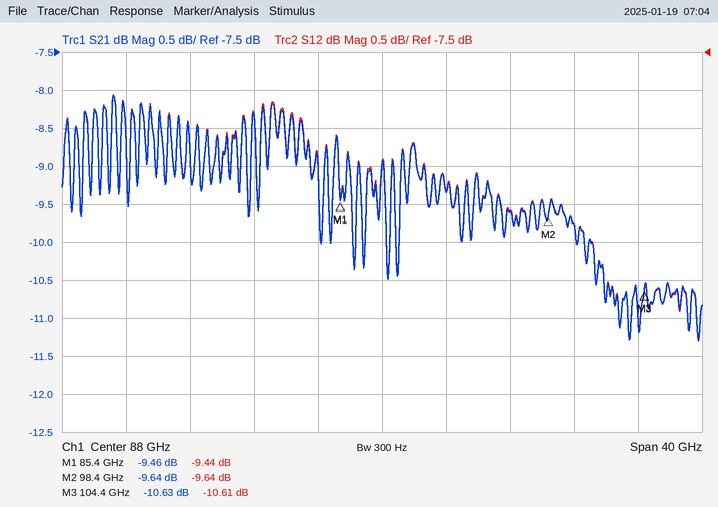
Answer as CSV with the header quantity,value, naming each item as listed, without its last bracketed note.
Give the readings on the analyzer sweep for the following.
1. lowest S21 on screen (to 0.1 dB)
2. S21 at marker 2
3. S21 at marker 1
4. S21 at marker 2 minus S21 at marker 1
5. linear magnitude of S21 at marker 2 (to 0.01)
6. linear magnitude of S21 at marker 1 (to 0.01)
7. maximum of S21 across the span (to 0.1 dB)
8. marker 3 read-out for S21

quantity,value
lowest S21 on screen,-11.3 dB
S21 at marker 2,-9.64 dB
S21 at marker 1,-9.46 dB
S21 at marker 2 minus S21 at marker 1,-0.18 dB
linear magnitude of S21 at marker 2,0.33
linear magnitude of S21 at marker 1,0.34
maximum of S21 across the span,-8.1 dB
marker 3 read-out for S21,-10.63 dB
